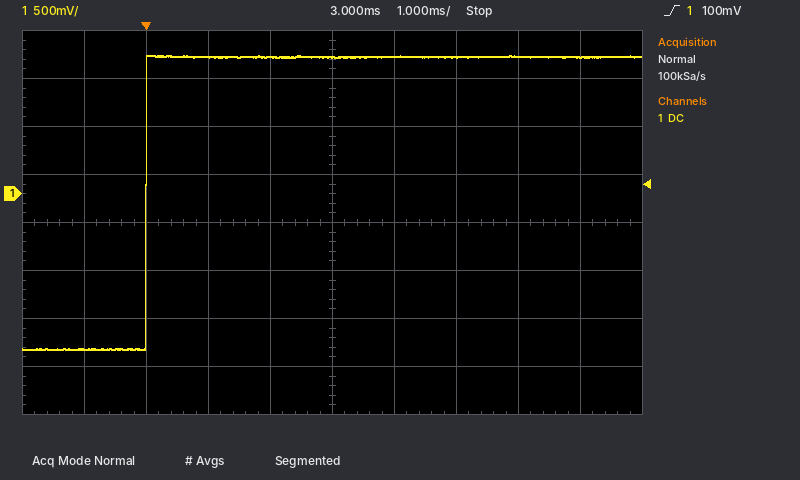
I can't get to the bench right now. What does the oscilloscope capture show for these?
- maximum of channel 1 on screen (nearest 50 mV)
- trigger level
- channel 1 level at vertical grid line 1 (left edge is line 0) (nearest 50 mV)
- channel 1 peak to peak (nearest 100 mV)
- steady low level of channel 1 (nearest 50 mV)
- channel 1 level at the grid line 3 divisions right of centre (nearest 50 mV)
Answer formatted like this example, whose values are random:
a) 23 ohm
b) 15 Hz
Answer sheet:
a) 1.45 V
b) 100 mV
c) -1.60 V
d) 3.10 V
e) -1.60 V
f) 1.45 V
